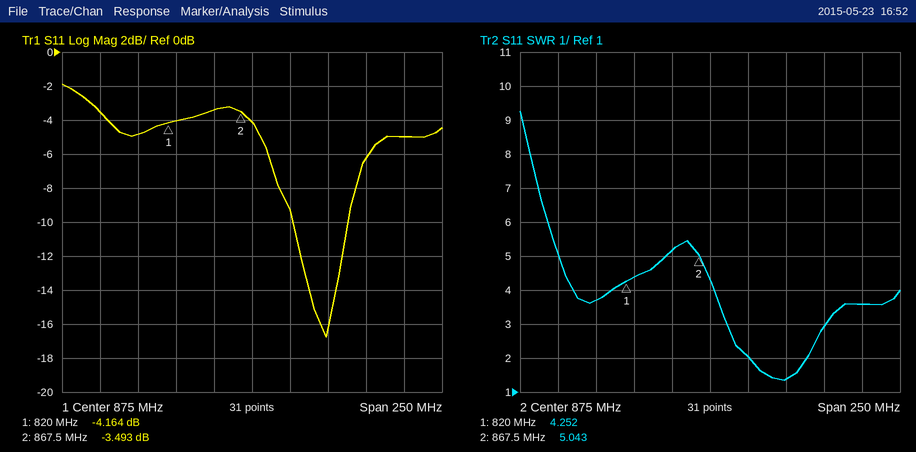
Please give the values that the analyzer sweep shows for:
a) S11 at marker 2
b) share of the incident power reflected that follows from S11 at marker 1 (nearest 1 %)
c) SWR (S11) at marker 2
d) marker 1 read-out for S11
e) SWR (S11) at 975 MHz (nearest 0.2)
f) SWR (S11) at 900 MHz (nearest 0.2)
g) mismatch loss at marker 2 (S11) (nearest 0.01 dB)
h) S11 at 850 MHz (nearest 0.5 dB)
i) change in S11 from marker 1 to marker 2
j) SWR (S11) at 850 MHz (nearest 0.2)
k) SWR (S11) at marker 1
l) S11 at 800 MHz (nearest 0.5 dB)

-3.493 dB
38 %
5.043
-4.164 dB
3.6
2.0
2.58 dB
-3.5 dB
0.671 dB
5.2
4.252
-5.0 dB
